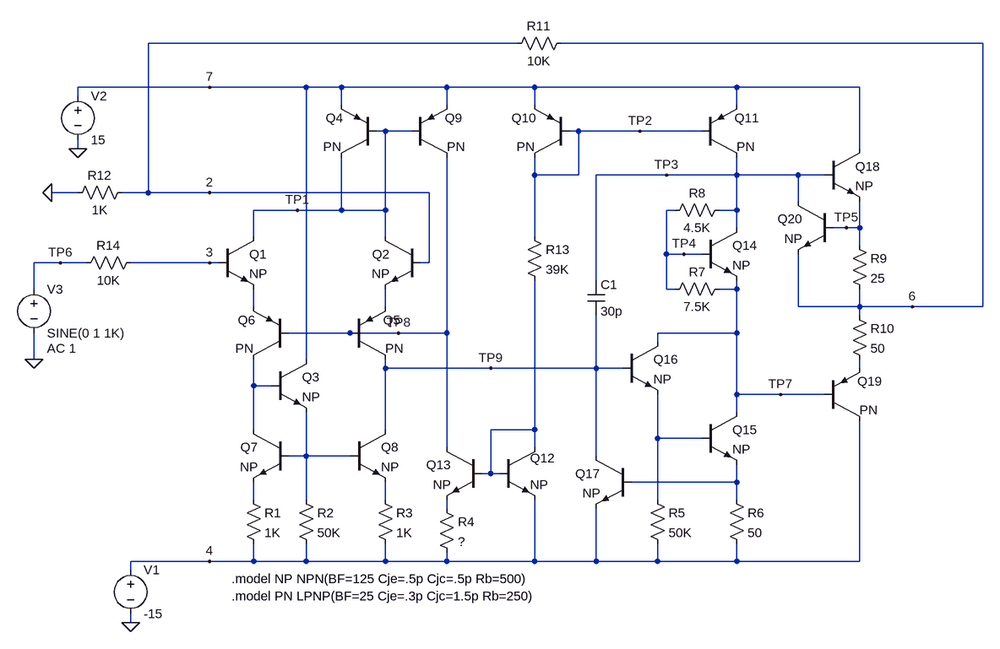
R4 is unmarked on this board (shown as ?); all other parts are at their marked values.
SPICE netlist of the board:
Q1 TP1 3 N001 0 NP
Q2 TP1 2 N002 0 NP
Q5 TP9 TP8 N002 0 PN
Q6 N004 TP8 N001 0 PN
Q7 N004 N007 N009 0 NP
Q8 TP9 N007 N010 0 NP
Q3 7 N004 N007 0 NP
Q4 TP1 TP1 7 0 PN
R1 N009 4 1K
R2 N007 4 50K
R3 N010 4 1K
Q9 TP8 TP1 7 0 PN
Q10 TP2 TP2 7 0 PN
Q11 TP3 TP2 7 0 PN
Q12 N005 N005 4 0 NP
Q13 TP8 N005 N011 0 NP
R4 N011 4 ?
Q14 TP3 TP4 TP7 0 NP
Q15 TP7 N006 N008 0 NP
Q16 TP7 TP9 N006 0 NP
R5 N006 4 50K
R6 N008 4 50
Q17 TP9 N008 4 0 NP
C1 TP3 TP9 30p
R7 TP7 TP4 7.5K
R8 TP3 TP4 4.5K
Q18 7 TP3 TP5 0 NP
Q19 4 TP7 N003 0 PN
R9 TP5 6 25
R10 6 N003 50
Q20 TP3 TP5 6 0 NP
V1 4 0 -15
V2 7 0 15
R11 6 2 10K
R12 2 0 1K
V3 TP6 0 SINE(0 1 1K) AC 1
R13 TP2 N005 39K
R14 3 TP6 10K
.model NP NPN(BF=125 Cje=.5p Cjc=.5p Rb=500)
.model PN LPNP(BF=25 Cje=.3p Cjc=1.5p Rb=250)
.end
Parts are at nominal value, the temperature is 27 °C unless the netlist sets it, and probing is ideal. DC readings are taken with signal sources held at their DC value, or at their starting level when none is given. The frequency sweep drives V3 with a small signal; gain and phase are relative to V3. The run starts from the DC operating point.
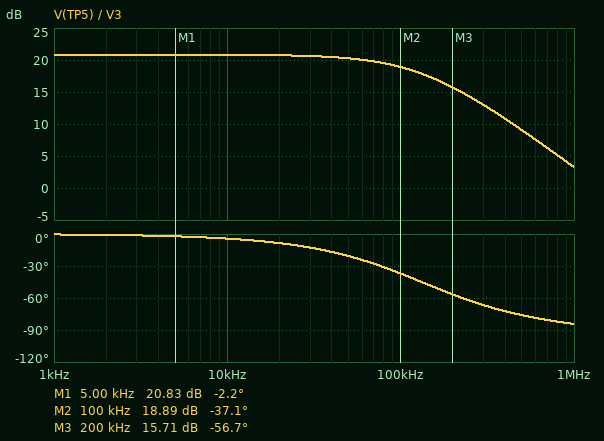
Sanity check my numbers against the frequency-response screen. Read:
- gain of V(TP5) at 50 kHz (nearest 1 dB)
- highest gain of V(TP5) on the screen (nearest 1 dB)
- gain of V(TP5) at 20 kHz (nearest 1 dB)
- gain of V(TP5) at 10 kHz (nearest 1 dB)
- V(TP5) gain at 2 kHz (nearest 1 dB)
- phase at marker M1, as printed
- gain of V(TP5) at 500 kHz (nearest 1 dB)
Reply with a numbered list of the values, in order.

1. 20 dB
2. 21 dB
3. 21 dB
4. 21 dB
5. 21 dB
6. -2.2 deg
7. 9 dB
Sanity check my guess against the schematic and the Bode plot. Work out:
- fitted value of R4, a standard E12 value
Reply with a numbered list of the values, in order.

1. 1.8 kΩ
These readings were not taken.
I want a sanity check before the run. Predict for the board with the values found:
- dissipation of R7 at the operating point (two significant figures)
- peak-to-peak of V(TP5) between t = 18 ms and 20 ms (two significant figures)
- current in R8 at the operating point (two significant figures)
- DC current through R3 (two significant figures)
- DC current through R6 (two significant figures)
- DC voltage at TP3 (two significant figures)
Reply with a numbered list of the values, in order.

1. 77 µW
2. 22 V
3. 110 µA
4. 21 µA
5. 660 µA
6. 600 mV
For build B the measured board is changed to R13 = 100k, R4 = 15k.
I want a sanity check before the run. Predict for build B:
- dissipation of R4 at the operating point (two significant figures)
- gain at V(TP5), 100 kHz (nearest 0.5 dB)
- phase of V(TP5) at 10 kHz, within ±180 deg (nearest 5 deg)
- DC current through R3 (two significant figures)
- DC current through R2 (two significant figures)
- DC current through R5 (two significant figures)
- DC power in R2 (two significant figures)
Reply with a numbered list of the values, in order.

1. 650 nW
2. 2.0 dB
3. -40 deg
4. 3.2 µA
5. 13 µA
6. 15 µA
7. 7.9 µW
